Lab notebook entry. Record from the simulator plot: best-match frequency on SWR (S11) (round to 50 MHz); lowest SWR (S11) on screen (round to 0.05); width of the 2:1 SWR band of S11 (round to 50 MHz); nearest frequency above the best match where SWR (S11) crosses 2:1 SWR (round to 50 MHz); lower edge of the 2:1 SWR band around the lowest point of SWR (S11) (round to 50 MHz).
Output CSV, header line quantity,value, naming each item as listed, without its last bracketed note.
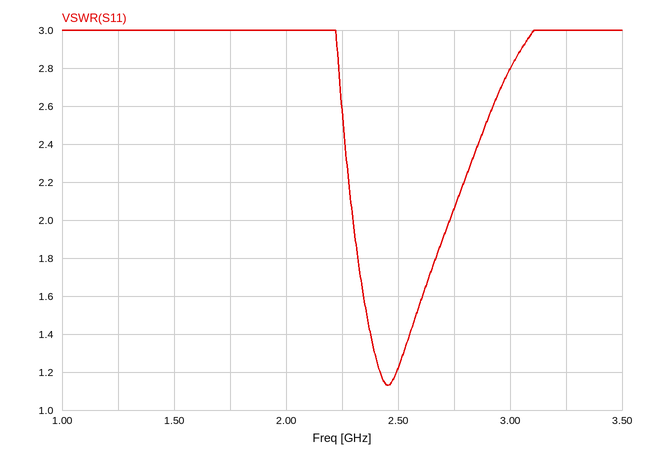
quantity,value
best-match frequency on SWR (S11),2.45 GHz
lowest SWR (S11) on screen,1.15
width of the 2:1 SWR band of S11,450 MHz
nearest frequency above the best match where SWR (S11) crosses 2:1 SWR,2.75 GHz
lower edge of the 2:1 SWR band around the lowest point of SWR (S11),2.30 GHz
